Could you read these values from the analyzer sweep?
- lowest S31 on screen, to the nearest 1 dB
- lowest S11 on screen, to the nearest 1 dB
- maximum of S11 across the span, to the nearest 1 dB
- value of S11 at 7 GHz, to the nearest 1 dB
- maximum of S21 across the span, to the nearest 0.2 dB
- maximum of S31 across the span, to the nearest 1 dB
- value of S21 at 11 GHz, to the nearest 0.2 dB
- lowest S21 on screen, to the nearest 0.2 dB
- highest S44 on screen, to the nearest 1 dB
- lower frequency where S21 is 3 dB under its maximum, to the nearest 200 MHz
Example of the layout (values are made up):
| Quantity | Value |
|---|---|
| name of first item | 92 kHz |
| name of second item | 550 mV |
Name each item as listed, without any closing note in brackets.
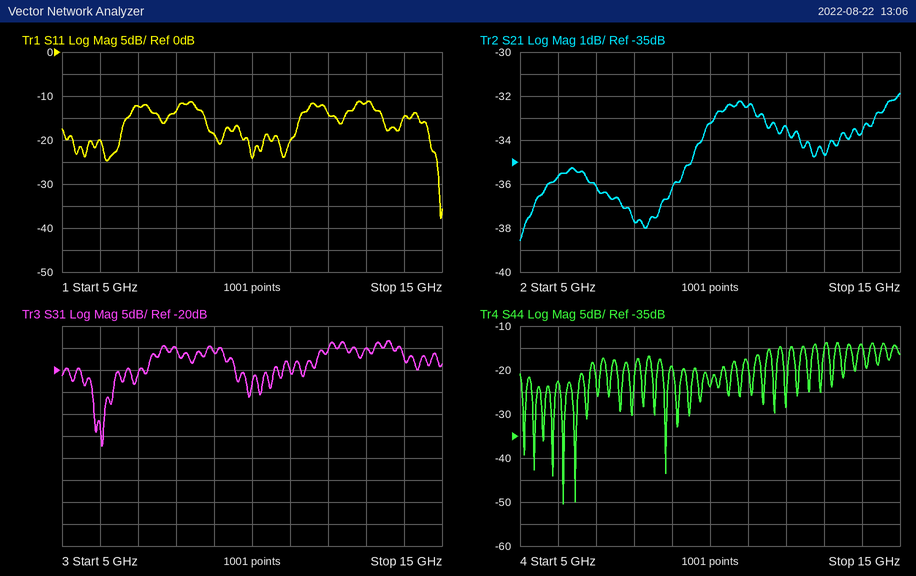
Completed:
| Quantity | Value |
|---|---|
| lowest S31 on screen, to the nearest 1 dB | -37 dB |
| lowest S11 on screen, to the nearest 1 dB | -38 dB |
| maximum of S11 across the span, to the nearest 1 dB | -11 dB |
| value of S11 at 7 GHz, to the nearest 1 dB | -12 dB |
| maximum of S21 across the span, to the nearest 0.2 dB | -31.8 dB |
| maximum of S31 across the span, to the nearest 1 dB | -13 dB |
| value of S21 at 11 GHz, to the nearest 0.2 dB | -32.4 dB |
| lowest S21 on screen, to the nearest 0.2 dB | -38.6 dB |
| highest S44 on screen, to the nearest 1 dB | -14 dB |
| lower frequency where S21 is 3 dB under its maximum, to the nearest 200 MHz | 9.6 GHz |
